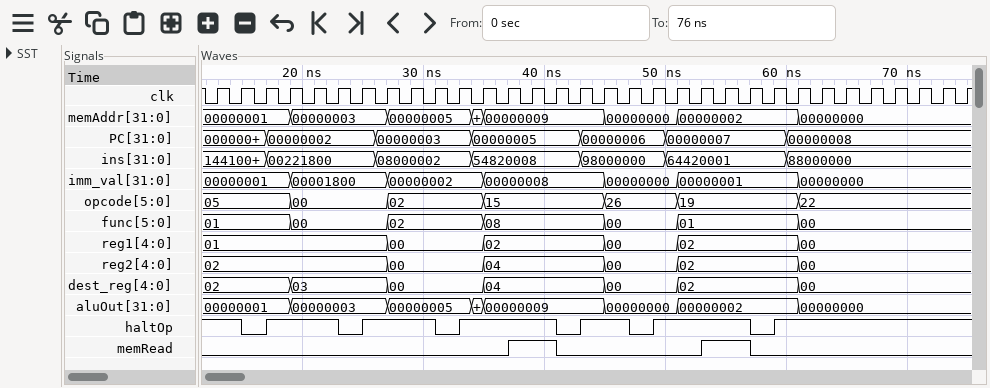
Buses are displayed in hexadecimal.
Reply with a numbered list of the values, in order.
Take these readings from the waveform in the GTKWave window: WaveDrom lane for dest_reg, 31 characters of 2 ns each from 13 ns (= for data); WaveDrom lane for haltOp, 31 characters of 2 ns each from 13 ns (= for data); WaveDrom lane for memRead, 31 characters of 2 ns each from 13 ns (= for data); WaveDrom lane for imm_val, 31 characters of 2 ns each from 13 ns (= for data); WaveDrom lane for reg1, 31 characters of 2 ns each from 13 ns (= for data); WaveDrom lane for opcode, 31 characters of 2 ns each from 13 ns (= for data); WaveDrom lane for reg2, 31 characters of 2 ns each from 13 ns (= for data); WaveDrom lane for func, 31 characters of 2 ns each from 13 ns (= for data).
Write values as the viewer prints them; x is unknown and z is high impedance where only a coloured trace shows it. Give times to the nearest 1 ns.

1. {name: 'dest_reg', wave: '=..=...=...=....=..=....=......', data: '02 03 00 04 00 02 00'}
2. {name: 'haltOp', wave: '101..01..01...01.01...01.......'}
3. {name: 'memRead', wave: '0...........1.0.....1.0........'}
4. {name: 'imm_val', wave: '=..=...=...=....=..=....=......', data: '00000001 00001800 00000002 00000008 00000000 00000001 00000000'}
5. {name: 'reg1', wave: '=......=...=....=..=....=......', data: '01 00 02 00 02 00'}
6. {name: 'opcode', wave: '=..=...=...=....=..=....=......', data: '05 00 02 15 26 19 22'}
7. {name: 'reg2', wave: '=......=...=....=..=....=......', data: '02 00 04 00 02 00'}
8. {name: 'func', wave: '=..=...=...=....=..=....=......', data: '01 00 02 08 00 01 00'}
